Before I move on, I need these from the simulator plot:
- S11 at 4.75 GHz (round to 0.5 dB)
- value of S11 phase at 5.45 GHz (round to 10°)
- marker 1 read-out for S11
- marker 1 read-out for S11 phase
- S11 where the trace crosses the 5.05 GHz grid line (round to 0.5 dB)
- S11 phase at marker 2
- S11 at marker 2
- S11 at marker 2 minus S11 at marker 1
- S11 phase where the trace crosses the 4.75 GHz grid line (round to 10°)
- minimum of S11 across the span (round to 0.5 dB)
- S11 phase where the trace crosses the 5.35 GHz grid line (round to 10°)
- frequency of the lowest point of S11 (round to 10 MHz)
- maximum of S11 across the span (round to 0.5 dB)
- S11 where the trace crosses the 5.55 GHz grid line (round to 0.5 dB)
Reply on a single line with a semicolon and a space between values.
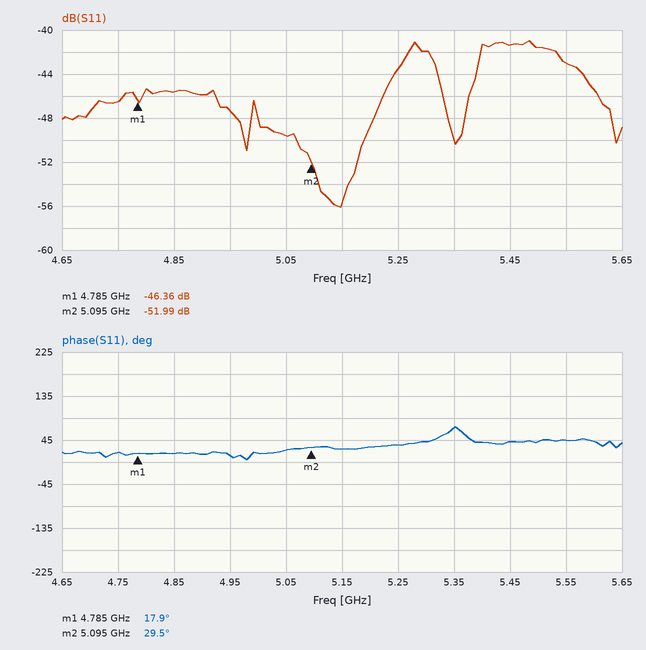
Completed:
-46.5 dB; 40°; -46.36 dB; 17.9°; -49.5 dB; 29.5°; -51.99 dB; -5.63 dB; 20°; -56.0 dB; 70°; 5.15 GHz; -41.0 dB; -43.0 dB
